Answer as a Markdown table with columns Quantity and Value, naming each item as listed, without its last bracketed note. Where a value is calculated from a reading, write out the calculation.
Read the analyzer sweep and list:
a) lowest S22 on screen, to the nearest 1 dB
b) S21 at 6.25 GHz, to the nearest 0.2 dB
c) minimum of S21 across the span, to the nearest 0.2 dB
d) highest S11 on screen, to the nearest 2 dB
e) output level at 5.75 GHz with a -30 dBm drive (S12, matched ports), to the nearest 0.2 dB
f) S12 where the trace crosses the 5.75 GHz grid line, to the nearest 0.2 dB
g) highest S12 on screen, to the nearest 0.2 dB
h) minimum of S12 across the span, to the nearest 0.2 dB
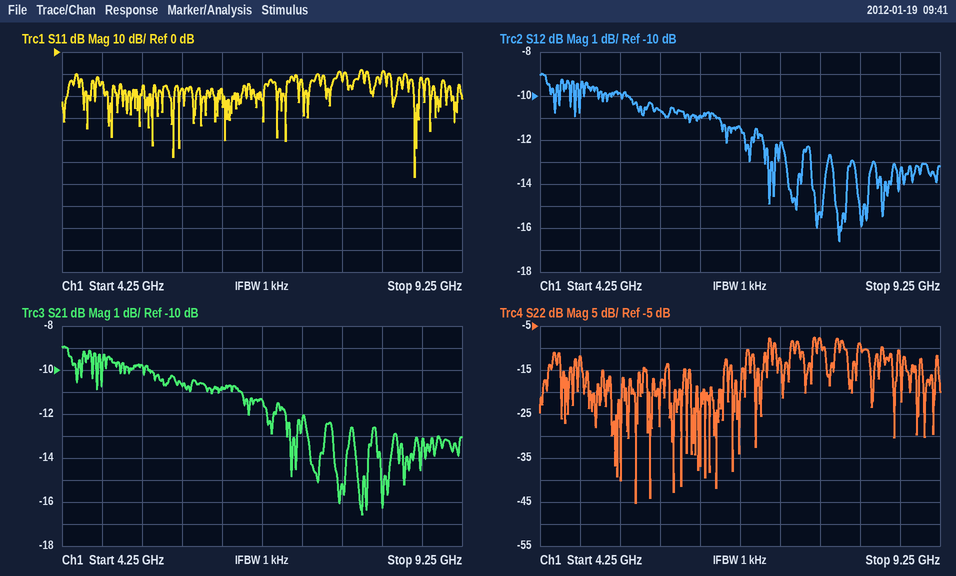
| Quantity | Value |
|---|---|
| lowest S22 on screen, to the nearest 1 dB | -45 dB |
| S21 at 6.25 GHz, to the nearest 0.2 dB | -10.8 dB |
| minimum of S21 across the span, to the nearest 0.2 dB | -16.6 dB |
| highest S11 on screen, to the nearest 2 dB | -8 dB |
| output level at 5.75 GHz with a -30 dBm drive (S12, matched ports), to the nearest 0.2 dB | -30 dBm + (-10.6 dB) = -40.6 dBm |
| S12 where the trace crosses the 5.75 GHz grid line, to the nearest 0.2 dB | -10.6 dB |
| highest S12 on screen, to the nearest 0.2 dB | -9.0 dB |
| minimum of S12 across the span, to the nearest 0.2 dB | -16.6 dB |
